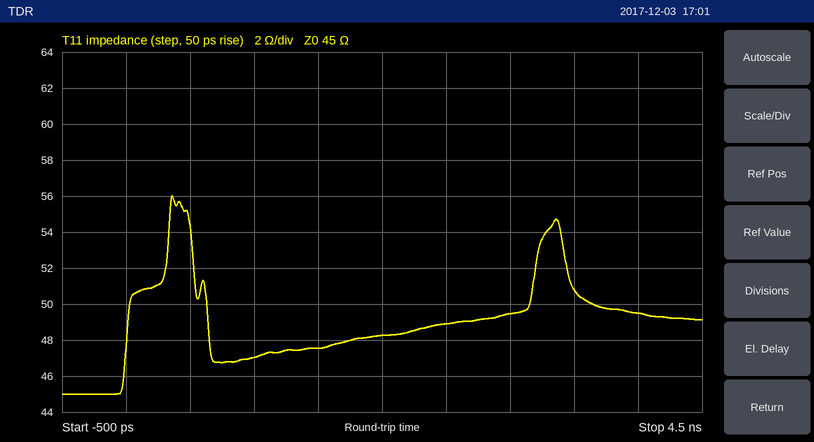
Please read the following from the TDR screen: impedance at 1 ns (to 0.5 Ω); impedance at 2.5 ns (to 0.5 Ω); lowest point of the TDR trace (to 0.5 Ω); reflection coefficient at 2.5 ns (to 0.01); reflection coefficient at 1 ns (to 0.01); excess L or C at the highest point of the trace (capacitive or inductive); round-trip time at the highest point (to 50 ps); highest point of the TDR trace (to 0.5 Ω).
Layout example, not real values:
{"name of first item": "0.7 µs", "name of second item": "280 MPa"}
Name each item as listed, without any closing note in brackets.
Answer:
{"impedance at 1 ns": "47.0 Ω", "impedance at 2.5 ns": "49.0 Ω", "lowest point of the TDR trace": "45.0 Ω", "reflection coefficient at 2.5 ns": "+0.04", "reflection coefficient at 1 ns": "+0.02", "excess L or C at the highest point of the trace": "inductive", "round-trip time at the highest point": "350 ps", "highest point of the TDR trace": "56.0 Ω"}
